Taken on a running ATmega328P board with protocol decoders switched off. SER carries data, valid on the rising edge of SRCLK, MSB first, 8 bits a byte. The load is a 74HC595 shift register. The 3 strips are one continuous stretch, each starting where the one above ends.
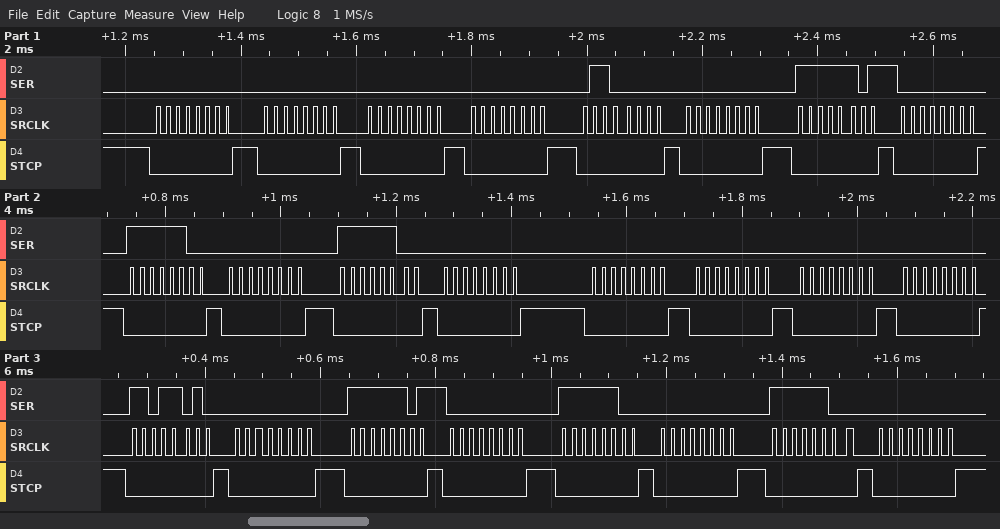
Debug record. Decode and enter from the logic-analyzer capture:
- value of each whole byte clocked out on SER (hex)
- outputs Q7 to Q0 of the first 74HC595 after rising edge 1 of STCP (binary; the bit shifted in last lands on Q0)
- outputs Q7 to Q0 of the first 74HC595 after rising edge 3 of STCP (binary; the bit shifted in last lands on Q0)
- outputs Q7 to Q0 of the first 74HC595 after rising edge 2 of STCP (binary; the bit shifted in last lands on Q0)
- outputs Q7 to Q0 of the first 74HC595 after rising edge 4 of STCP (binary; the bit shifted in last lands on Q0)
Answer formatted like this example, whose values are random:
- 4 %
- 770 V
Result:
- 00 00 00 00 60 00 FD 00 FC 00 FC 00 00 00 00 00 DA 00 FD 00 FC 00 FC 00
- 00000000
- 00000000
- 00000000
- 00000000
